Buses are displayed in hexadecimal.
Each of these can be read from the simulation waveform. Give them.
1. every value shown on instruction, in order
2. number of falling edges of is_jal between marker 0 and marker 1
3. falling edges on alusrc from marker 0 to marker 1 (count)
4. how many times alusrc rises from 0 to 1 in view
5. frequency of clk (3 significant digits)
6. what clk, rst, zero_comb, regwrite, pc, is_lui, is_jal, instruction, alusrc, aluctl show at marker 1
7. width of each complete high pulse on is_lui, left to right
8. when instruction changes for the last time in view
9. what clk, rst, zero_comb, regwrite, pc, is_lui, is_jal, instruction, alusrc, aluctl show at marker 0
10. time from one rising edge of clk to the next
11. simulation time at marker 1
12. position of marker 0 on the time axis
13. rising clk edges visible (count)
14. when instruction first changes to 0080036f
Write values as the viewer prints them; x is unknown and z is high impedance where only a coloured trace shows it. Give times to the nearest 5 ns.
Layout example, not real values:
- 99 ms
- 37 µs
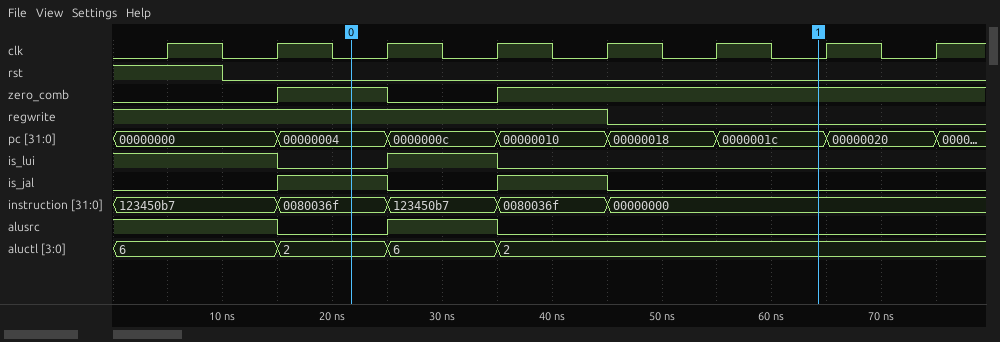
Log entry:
- 123450b7, 0080036f, 123450b7, 0080036f, 00000000
- 2
- 1
- 1
- 100 MHz
- clk=0, rst=0, zero_comb=1, regwrite=0, pc=0000001c, is_lui=0, is_jal=0, instruction=00000000, alusrc=0, aluctl=2
- 10 ns
- 45 ns
- clk=0, rst=0, zero_comb=1, regwrite=1, pc=00000004, is_lui=0, is_jal=1, instruction=0080036f, alusrc=0, aluctl=2
- 10 ns
- 65 ns
- 20 ns
- 8
- 15 ns
